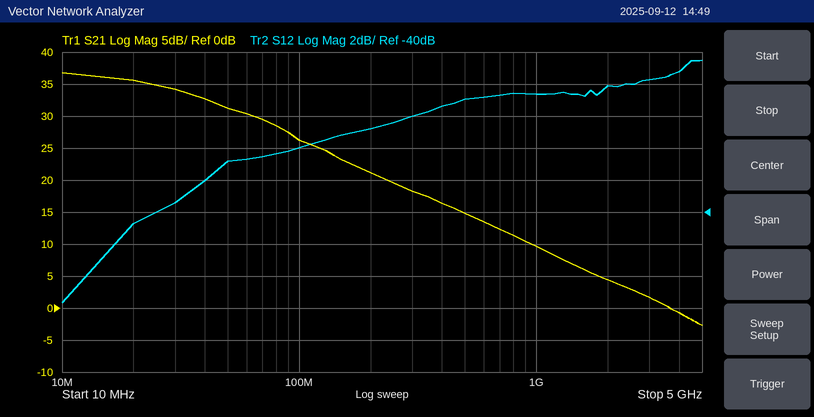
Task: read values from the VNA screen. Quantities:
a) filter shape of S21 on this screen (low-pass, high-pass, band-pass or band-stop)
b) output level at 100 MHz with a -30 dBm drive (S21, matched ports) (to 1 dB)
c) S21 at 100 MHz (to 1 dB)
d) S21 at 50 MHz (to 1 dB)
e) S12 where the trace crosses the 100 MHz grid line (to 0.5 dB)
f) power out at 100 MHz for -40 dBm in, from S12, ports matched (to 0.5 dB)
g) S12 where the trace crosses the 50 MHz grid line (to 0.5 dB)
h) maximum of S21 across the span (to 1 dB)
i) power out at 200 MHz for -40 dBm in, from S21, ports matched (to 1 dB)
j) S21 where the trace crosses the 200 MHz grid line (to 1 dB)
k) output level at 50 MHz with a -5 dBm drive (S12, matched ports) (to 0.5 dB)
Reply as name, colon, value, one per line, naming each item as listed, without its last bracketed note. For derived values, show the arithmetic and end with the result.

filter shape of S21 on this screen: low-pass
output level at 100 MHz with a -30 dBm drive (S21, matched ports): -30 dBm + (26 dB) = -4 dBm
S21 at 100 MHz: 26 dB
S21 at 50 MHz: 31 dB
S12 where the trace crosses the 100 MHz grid line: -36.0 dB
power out at 100 MHz for -40 dBm in, from S12, ports matched: -40 dBm + (-36.0 dB) = -76.0 dBm
S12 where the trace crosses the 50 MHz grid line: -37.0 dB
maximum of S21 across the span: 37 dB
power out at 200 MHz for -40 dBm in, from S21, ports matched: -40 dBm + (21 dB) = -19 dBm
S21 where the trace crosses the 200 MHz grid line: 21 dB
output level at 50 MHz with a -5 dBm drive (S12, matched ports): -5 dBm + (-37.0 dB) = -42.0 dBm
